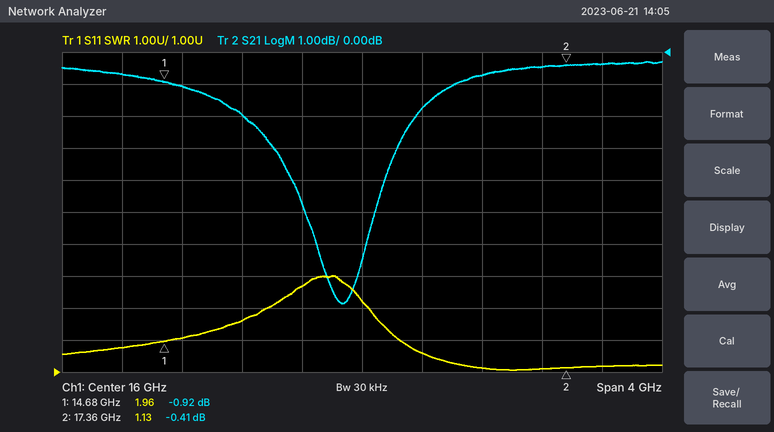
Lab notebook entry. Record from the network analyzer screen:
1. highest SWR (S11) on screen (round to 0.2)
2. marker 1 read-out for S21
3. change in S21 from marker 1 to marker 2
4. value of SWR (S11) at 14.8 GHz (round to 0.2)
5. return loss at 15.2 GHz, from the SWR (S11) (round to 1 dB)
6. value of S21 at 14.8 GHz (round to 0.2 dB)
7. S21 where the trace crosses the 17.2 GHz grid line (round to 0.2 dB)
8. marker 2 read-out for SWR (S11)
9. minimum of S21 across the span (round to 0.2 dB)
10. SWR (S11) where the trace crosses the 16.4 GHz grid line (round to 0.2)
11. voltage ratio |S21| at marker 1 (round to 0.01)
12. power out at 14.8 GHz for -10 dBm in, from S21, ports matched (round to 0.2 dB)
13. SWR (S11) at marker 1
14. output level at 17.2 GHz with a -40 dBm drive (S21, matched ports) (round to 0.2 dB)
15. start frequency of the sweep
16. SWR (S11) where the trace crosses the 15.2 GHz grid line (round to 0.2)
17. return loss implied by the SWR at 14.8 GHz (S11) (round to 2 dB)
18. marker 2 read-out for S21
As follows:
4.0
-0.92 dB
0.51 dB
2.0
7 dB
-1.0 dB
-0.4 dB
1.13
-7.8 dB
1.6
0.90
-11.0 dBm
1.96
-40.4 dBm
14 GHz
2.6
10 dB
-0.41 dB
